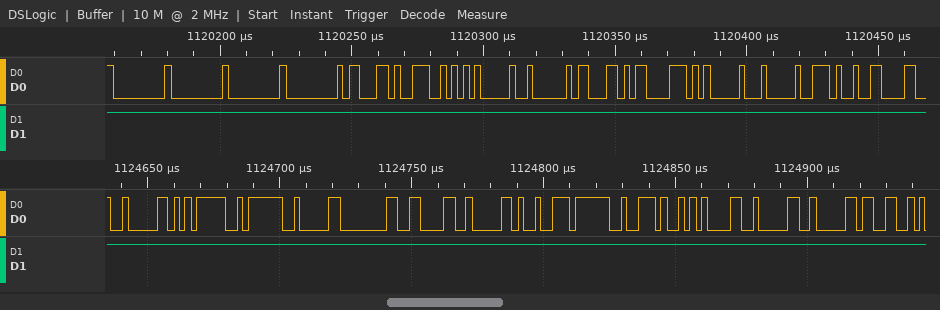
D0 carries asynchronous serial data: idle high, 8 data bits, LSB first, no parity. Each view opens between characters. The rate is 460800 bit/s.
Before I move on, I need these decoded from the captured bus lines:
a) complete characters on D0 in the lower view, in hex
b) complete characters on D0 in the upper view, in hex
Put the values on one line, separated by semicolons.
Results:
82, F5, FA, 82, 80, 86, 82, C9, 3F, 2E, 85, 82, 82, 33; 00, 00, 00, 00, 63, 4E, 05, 02, 63, C3, 05, 04, 2E, 86
